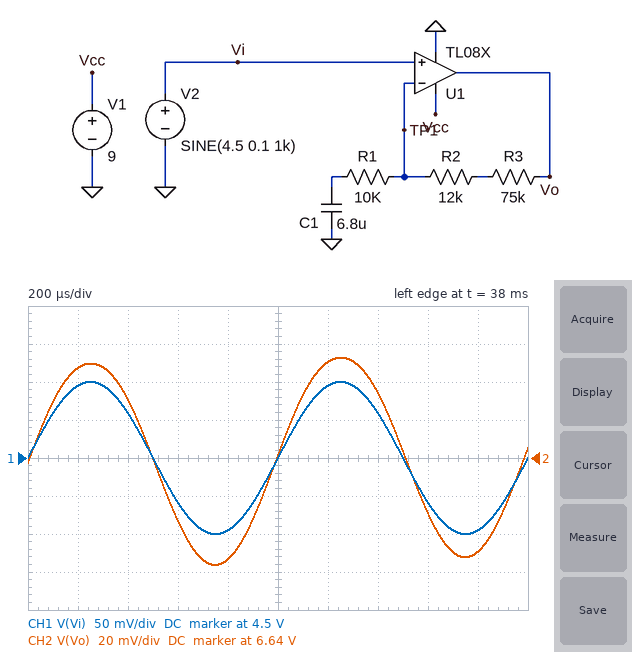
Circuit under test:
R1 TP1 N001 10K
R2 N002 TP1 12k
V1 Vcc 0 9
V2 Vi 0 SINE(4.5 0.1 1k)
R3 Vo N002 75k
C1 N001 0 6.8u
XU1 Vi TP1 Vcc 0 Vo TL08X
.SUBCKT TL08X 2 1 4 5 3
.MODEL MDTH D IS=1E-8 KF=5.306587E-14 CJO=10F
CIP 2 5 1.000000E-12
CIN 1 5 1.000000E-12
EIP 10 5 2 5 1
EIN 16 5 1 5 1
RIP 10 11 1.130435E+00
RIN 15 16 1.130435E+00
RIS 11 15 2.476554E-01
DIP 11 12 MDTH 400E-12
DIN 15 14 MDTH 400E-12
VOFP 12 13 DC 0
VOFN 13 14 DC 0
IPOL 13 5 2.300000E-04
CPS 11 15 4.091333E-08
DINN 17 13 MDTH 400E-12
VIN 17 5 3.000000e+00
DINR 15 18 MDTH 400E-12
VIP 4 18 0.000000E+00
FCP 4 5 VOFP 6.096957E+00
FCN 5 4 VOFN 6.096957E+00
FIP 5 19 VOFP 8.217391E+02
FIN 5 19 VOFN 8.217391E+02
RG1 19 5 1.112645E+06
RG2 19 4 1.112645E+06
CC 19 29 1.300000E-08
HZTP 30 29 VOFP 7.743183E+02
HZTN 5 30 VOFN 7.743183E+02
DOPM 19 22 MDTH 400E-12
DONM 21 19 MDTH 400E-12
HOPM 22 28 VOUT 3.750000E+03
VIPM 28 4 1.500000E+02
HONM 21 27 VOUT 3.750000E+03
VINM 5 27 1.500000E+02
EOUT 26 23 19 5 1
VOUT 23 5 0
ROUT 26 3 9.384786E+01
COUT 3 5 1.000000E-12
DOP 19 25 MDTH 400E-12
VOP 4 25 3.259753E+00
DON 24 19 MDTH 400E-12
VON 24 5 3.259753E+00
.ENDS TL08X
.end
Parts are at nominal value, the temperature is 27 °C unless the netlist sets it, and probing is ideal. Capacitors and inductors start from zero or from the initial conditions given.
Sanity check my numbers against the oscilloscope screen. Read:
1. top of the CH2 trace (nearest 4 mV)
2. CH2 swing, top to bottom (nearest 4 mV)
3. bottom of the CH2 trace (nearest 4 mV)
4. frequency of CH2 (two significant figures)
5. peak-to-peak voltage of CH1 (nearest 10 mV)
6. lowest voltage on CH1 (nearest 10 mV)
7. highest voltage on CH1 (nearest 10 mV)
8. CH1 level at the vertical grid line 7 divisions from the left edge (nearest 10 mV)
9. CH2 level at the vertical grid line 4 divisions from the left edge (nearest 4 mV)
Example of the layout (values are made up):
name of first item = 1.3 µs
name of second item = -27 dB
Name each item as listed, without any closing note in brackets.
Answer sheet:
top of the CH2 trace = 6.692 V
CH2 swing, top to bottom = 108 mV
bottom of the CH2 trace = 6.584 V
frequency of CH2 = 1.0 kHz
peak-to-peak voltage of CH1 = 200 mV
lowest voltage on CH1 = 4.40 V
highest voltage on CH1 = 4.60 V
CH1 level at the vertical grid line 7 divisions from the left edge = 4.56 V
CH2 level at the vertical grid line 4 divisions from the left edge = 6.588 V
